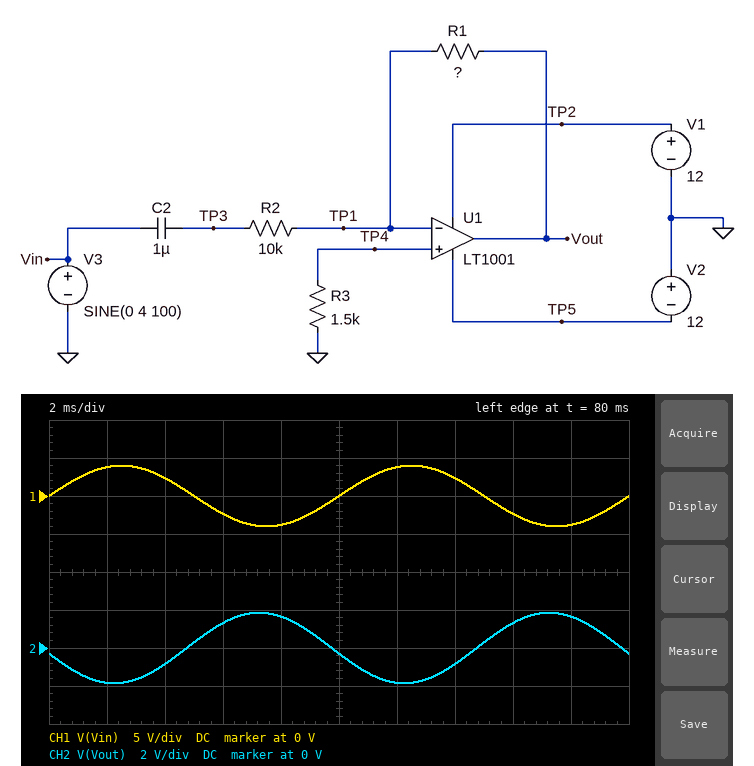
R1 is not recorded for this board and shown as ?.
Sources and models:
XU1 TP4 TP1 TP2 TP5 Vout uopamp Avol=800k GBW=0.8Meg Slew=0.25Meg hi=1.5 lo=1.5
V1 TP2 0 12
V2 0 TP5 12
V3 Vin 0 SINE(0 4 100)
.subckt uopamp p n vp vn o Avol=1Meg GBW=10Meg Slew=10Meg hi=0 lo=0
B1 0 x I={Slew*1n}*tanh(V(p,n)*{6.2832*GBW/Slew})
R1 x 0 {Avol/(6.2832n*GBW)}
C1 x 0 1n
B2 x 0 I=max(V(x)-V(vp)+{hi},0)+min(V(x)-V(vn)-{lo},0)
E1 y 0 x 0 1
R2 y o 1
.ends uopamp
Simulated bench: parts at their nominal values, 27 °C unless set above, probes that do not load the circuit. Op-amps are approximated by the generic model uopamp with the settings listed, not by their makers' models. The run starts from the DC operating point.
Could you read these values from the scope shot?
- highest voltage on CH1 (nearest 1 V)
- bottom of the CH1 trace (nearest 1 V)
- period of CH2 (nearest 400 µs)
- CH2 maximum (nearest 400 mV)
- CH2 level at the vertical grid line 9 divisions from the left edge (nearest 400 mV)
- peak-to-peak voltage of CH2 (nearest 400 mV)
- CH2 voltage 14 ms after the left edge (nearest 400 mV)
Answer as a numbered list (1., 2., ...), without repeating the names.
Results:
1. 4 V
2. -4 V
3. 10.0 ms
4. 2.0 V
5. 1.6 V
6. 3.6 V
7. -800 mV
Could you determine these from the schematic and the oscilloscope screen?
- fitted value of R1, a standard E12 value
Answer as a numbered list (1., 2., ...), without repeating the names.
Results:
1. 4.7 kΩ
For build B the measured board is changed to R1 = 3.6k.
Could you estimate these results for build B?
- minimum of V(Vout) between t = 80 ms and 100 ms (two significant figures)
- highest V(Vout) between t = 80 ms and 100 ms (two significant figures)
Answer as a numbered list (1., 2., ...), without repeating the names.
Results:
1. -1.4 V
2. 1.4 V
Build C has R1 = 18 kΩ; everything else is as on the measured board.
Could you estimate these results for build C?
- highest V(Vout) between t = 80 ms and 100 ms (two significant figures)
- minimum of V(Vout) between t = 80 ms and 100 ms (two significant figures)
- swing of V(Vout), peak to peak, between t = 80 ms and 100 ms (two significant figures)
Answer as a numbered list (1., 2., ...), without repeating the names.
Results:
1. 7.1 V
2. -7.1 V
3. 14 V
